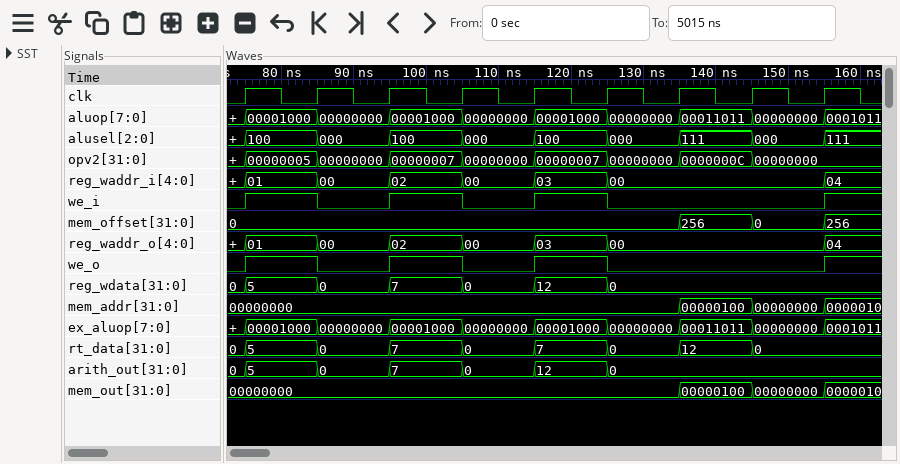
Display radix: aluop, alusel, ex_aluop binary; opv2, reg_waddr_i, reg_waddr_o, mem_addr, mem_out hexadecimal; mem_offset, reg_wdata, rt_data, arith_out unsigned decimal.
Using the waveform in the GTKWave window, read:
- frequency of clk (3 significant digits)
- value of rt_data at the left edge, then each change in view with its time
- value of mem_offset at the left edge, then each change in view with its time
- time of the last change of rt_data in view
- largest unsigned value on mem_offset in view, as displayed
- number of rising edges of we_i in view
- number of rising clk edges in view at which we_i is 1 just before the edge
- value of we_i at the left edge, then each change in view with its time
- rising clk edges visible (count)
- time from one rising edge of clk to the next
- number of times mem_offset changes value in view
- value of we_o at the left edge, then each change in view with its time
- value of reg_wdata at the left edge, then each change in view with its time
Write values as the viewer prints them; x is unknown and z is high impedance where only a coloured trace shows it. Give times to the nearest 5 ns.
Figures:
100 MHz
0, 5 at 75 ns, 0 at 85 ns, 7 at 95 ns, 0 at 105 ns, 7 at 115 ns, 0 at 125 ns, 12 at 135 ns, 0 at 145 ns
0, 256 at 135 ns, 0 at 145 ns, 256 at 155 ns
145 ns
256
4
3
0, 1 at 75 ns, 0 at 85 ns, 1 at 95 ns, 0 at 105 ns, 1 at 115 ns, 0 at 125 ns, 1 at 155 ns
9
10 ns
3
0, 1 at 75 ns, 0 at 85 ns, 1 at 95 ns, 0 at 105 ns, 1 at 115 ns, 0 at 125 ns, 1 at 155 ns
0, 5 at 75 ns, 0 at 85 ns, 7 at 95 ns, 0 at 105 ns, 12 at 115 ns, 0 at 125 ns
